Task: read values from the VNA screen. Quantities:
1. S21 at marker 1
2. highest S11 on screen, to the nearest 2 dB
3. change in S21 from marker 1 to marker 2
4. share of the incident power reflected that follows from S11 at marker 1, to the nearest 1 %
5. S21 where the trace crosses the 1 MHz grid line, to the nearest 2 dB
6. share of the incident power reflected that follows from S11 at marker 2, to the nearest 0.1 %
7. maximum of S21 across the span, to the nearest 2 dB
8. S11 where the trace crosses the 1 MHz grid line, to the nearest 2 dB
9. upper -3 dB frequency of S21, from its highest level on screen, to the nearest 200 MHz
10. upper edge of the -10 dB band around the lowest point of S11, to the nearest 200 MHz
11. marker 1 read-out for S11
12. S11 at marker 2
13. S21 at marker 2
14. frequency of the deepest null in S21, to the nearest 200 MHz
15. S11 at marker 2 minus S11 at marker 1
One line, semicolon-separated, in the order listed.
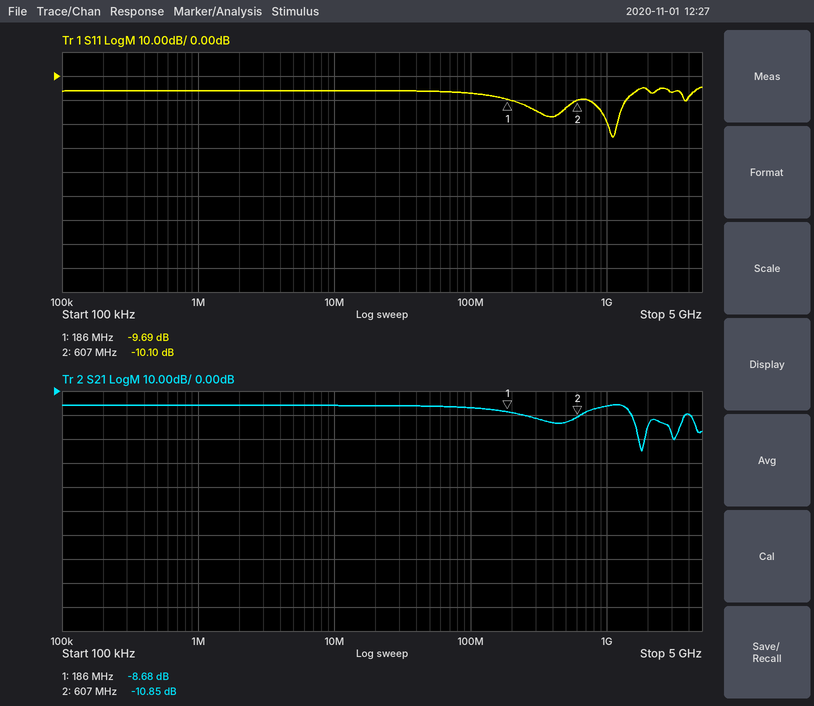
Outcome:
-8.68 dB; -4 dB; -2.17 dB; 11 %; -6 dB; 9.8 %; -6 dB; -6 dB; 1.4 GHz; 1.4 GHz; -9.69 dB; -10.10 dB; -10.85 dB; 1.8 GHz; -0.41 dB
